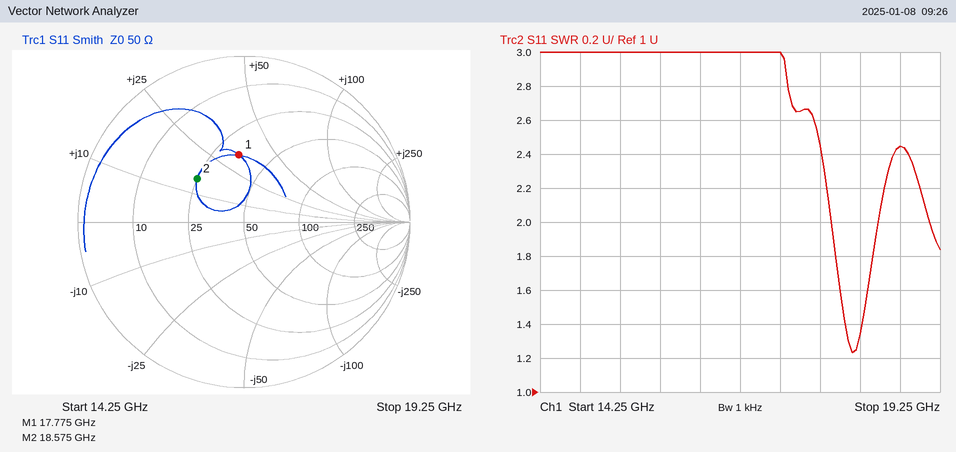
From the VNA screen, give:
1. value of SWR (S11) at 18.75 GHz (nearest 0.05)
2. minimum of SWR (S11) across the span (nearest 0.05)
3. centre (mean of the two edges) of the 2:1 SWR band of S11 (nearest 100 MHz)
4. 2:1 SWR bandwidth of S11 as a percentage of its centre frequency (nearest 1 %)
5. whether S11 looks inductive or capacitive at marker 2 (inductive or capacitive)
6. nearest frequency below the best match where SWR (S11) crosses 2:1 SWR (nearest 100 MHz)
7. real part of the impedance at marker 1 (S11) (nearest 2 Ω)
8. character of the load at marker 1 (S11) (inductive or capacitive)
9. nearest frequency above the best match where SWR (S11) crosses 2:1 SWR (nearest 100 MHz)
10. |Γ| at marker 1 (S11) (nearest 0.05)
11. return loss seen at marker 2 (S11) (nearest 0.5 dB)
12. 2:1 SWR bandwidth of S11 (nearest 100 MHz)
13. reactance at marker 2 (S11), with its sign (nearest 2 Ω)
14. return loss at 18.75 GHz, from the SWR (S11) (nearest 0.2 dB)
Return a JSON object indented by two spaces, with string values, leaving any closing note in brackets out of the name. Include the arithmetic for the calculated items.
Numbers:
{
  "value of SWR (S11) at 18.75 GHz": "2.45",
  "minimum of SWR (S11) across the span": "1.25",
  "centre (mean of the two edges) of the 2:1 SWR band of S11": "18.2 GHz",
  "2:1 SWR bandwidth of S11 as a percentage of its centre frequency": "600 MHz / 18.2 GHz ≈ 3 %",
  "whether S11 looks inductive or capacitive at marker 2": "inductive",
  "nearest frequency below the best match where SWR (S11) crosses 2:1 SWR": "17.9 GHz",
  "real part of the impedance at marker 1 (S11)": "34 Ω",
  "character of the load at marker 1 (S11)": "inductive",
  "nearest frequency above the best match where SWR (S11) crosses 2:1 SWR": "18.5 GHz",
  "|Γ| at marker 1 (S11)": "0.40",
  "return loss seen at marker 2 (S11)": "8.5 dB",
  "2:1 SWR bandwidth of S11": "18.5 GHz − 17.9 GHz = 600 MHz",
  "reactance at marker 2 (S11), with its sign": "+16 Ω",
  "return loss at 18.75 GHz, from the SWR (S11)": "−20 log10((2.45 − 1)/(2.45 + 1)) ≈ 7.53 dB, so 7.6 dB to the nearest 0.2 dB"
}
